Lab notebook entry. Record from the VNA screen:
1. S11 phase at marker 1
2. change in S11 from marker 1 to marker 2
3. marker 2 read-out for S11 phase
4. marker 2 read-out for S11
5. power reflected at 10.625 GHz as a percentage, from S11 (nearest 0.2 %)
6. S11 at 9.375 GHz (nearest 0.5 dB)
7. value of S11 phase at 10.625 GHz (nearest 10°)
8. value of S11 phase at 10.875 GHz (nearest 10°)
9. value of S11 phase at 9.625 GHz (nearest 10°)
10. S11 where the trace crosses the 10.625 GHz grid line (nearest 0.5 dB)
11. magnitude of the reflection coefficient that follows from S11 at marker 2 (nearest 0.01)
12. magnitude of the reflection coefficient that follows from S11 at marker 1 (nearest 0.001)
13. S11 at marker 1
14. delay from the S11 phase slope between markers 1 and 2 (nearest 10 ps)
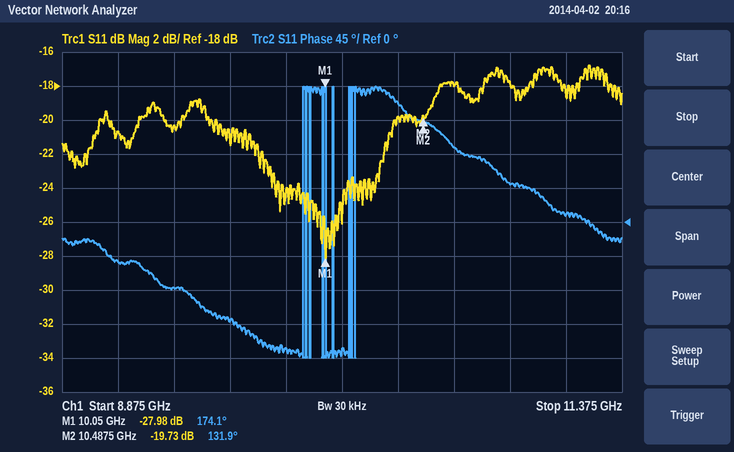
174.1°
8.25 dB
131.9°
-19.73 dB
1.6 %
-20.5 dB
100°
50°
-130°
-18.0 dB
0.10
0.040
-27.98 dB
270 ps
